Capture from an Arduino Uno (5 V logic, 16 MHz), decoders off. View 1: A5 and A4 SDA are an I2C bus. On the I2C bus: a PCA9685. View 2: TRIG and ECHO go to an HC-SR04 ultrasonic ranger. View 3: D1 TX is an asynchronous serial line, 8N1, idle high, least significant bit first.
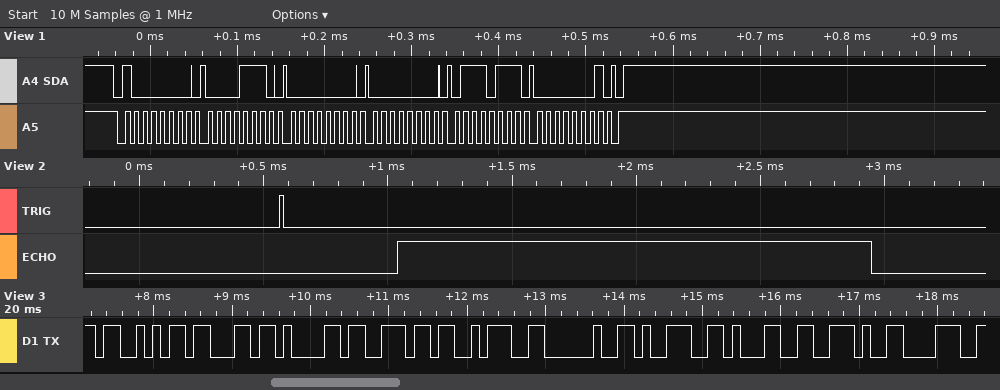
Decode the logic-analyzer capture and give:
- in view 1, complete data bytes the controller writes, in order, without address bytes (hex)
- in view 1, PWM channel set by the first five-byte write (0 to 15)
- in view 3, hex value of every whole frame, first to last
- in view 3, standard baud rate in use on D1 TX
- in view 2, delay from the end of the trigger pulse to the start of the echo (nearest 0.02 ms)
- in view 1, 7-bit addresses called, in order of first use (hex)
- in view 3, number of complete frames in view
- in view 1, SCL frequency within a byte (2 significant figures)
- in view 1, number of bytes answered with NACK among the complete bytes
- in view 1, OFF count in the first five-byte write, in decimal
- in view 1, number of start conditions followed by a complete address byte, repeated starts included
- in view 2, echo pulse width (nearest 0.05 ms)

0E 00 00 77 01
2
0x53 0x63 0x61 0x6E 0x3A 0x20 0x39 0x31 0x2E 0x38
9600 baud
0.46 ms
0x40
10
100 kHz
0
375
1
1.90 ms
